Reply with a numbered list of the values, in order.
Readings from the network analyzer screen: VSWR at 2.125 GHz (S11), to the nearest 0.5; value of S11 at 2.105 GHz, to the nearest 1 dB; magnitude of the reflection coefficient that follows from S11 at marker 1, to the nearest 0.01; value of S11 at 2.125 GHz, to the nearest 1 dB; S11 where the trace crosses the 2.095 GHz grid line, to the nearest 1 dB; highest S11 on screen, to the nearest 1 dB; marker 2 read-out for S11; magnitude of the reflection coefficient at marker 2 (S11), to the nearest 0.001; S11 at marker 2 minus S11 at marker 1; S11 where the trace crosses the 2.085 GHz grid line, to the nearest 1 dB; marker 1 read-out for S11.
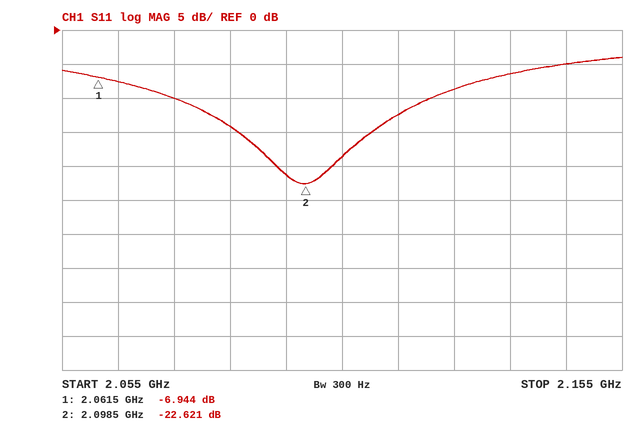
1. 2.0
2. -19 dB
3. 0.45
4. -9 dB
5. -21 dB
6. -4 dB
7. -22.621 dB
8. 0.074
9. -15.677 dB
10. -14 dB
11. -6.944 dB
